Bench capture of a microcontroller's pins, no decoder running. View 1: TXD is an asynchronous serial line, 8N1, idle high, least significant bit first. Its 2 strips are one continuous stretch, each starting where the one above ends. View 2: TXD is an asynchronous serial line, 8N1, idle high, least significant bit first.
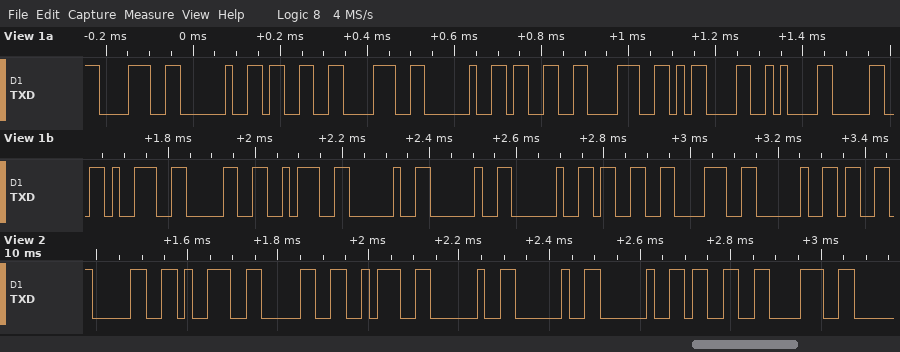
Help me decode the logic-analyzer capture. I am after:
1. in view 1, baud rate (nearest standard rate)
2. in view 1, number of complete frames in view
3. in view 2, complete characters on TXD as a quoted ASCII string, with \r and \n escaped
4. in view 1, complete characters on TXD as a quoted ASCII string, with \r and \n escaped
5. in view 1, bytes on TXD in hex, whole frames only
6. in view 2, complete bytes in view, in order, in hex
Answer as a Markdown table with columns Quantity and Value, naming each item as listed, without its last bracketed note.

| Quantity | Value |
|---|---|
| in view 1, baud rate | 57600 baud |
| in view 1, number of complete frames in view | 19 |
| in view 2, complete characters on TXD as a quoted ASCII string, with \r and \n escaped | "090:   38" |
| in view 1, complete characters on TXD as a quoted ASCII string, with \r and \n escaped | "8 38 38\r\n090:   38 " |
| in view 1, bytes on TXD in hex, whole frames only | 38 20 33 38 20 33 38 0D 0A 30 39 30 3A 20 20 20 33 38 20 |
| in view 2, complete bytes in view, in order, in hex | 30 39 30 3A 20 20 20 33 38 |
